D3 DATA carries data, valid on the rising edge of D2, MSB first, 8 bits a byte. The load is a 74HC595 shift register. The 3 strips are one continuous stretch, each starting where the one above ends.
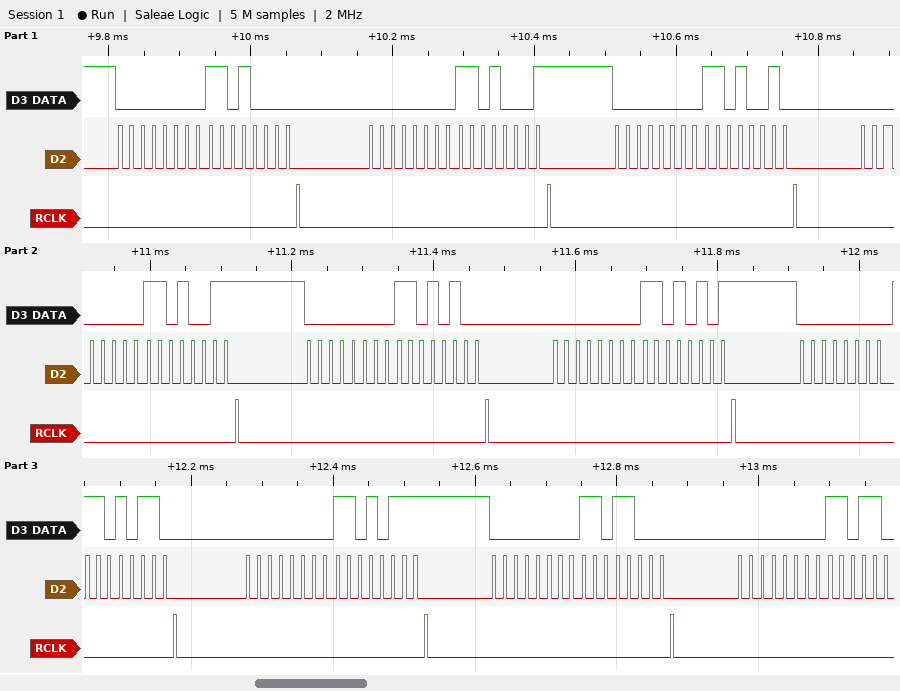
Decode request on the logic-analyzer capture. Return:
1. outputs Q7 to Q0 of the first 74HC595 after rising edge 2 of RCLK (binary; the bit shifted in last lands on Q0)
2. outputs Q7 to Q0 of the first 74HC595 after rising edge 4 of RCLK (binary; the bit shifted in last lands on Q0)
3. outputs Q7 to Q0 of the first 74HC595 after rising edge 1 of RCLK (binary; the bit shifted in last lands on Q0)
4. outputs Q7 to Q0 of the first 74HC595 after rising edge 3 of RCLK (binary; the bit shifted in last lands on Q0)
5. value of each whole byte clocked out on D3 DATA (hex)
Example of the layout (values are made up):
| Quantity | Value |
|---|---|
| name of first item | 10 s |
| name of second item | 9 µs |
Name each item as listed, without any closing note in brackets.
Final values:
| Quantity | Value |
|---|---|
| outputs Q7 to Q0 of the first 74HC595 after rising edge 2 of RCLK | 11010001 |
| outputs Q7 to Q0 of the first 74HC595 after rising edge 4 of RCLK | 11010011 |
| outputs Q7 to Q0 of the first 74HC595 after rising edge 1 of RCLK | 11010000 |
| outputs Q7 to Q0 of the first 74HC595 after rising edge 3 of RCLK | 11010010 |
| value of each whole byte clocked out on D3 DATA | 0x00 0xD0 0x00 0xD1 0x00 0xD2 0x00 0xD3 0x00 0xD4 0x00 0xD5 0x00 0xD6 0x00 0xD7 0x00 0xD8 0x00 |
